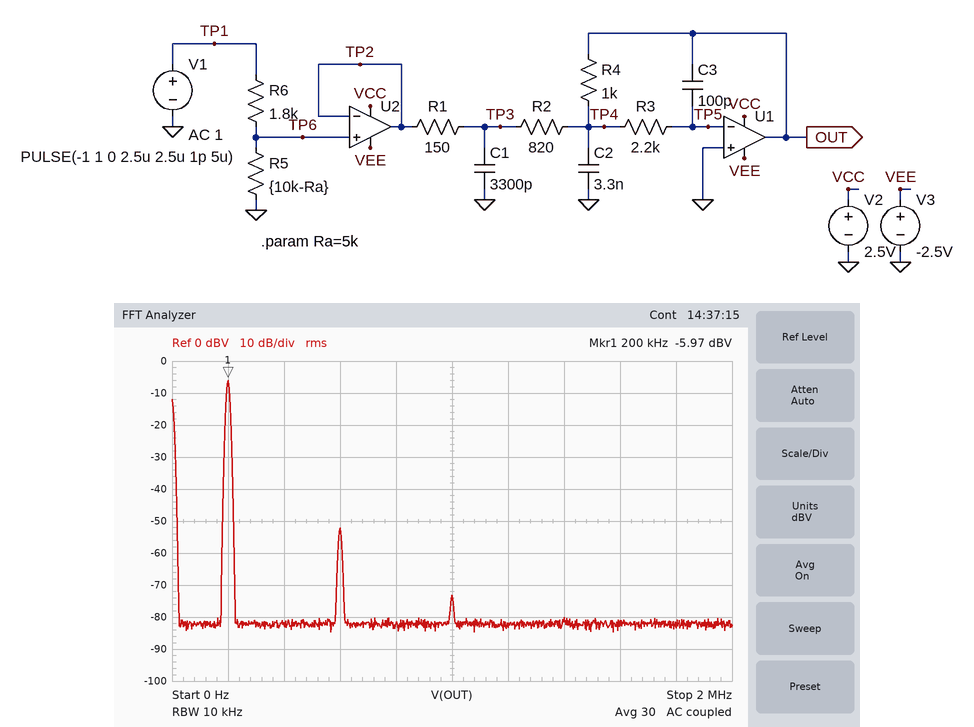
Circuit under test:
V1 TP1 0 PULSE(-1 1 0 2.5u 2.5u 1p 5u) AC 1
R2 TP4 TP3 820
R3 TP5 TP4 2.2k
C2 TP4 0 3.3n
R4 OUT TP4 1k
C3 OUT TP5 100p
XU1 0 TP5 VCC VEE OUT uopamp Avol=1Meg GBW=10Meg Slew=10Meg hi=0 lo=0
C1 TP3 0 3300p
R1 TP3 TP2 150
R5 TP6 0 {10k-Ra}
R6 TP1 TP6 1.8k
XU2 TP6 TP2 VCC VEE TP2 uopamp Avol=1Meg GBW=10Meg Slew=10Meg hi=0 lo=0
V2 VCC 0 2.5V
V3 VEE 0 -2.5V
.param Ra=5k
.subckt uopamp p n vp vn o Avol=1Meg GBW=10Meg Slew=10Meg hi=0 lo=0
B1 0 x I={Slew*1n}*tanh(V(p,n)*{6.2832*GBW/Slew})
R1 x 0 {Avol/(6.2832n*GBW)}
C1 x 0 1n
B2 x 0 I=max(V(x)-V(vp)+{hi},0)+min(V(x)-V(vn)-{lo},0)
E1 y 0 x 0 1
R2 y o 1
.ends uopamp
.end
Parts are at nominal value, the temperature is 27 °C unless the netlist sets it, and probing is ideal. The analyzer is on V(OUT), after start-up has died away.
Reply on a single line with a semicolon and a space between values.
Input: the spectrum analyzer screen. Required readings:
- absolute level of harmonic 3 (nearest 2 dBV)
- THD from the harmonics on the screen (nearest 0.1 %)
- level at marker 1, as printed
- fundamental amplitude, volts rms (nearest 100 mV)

-52 dBV; 0.5 %; -5.97 dBV; 500 mV
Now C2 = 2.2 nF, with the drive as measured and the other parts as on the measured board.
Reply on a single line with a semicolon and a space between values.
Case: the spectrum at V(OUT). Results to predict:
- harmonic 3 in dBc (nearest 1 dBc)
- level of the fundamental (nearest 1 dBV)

-43 dBc; -6 dBV
